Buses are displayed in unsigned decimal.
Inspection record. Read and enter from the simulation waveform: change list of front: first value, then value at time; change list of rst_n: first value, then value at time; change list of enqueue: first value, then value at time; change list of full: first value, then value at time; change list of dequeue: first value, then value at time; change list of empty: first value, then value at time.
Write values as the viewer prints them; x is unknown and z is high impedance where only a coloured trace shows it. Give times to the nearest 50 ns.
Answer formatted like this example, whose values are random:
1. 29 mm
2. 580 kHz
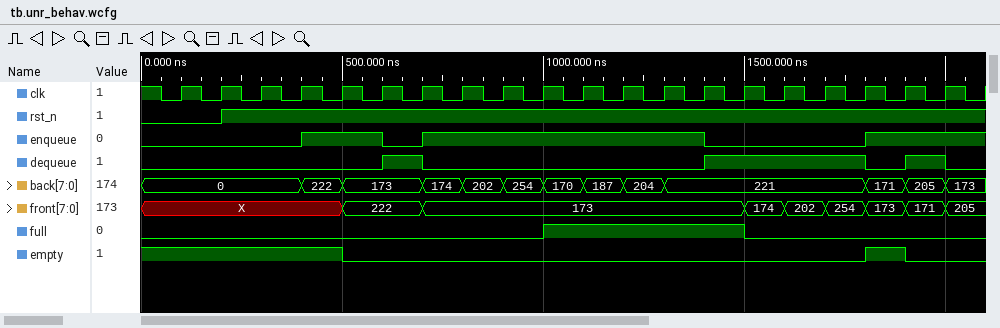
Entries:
1. X, 222 at 500 ns, 173 at 700 ns, 174 at 1500 ns, 202 at 1600 ns, 254 at 1700 ns, 173 at 1800 ns, 171 at 1900 ns, 205 at 2000 ns
2. 0, 1 at 200 ns
3. 0, 1 at 400 ns, 0 at 600 ns, 1 at 700 ns, 0 at 1400 ns, 1 at 1800 ns
4. 0, 1 at 1000 ns, 0 at 1500 ns
5. 0, 1 at 600 ns, 0 at 700 ns, 1 at 1400 ns, 0 at 1800 ns, 1 at 1900 ns, 0 at 2000 ns
6. 1, 0 at 500 ns, 1 at 1800 ns, 0 at 1900 ns
